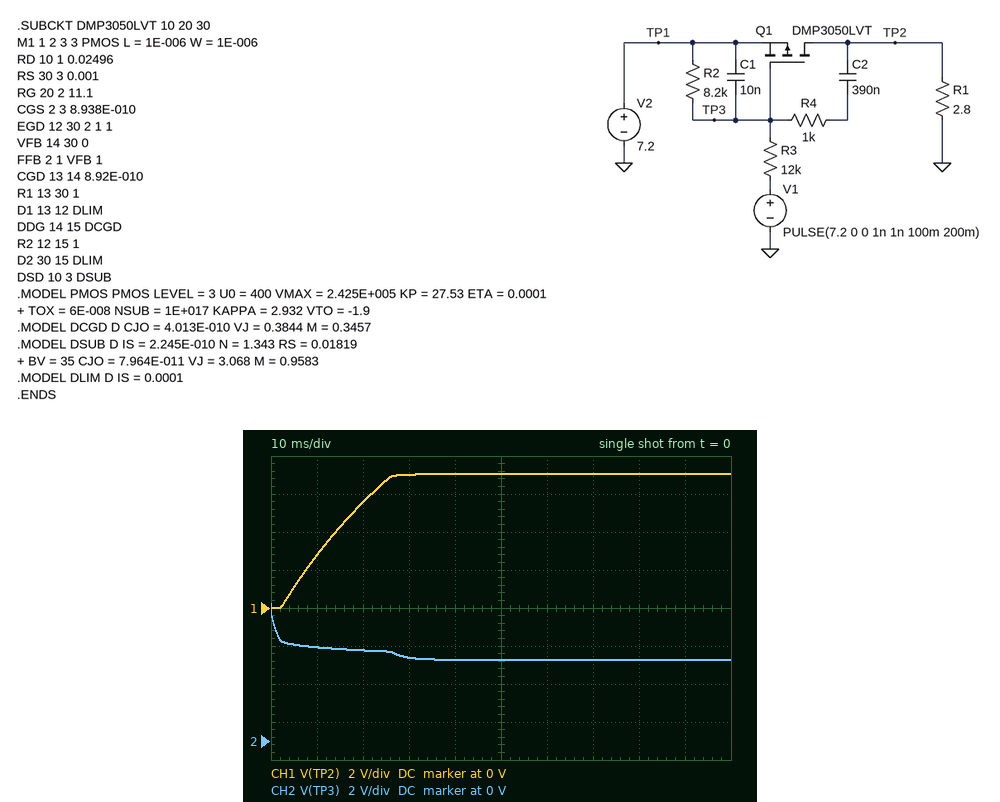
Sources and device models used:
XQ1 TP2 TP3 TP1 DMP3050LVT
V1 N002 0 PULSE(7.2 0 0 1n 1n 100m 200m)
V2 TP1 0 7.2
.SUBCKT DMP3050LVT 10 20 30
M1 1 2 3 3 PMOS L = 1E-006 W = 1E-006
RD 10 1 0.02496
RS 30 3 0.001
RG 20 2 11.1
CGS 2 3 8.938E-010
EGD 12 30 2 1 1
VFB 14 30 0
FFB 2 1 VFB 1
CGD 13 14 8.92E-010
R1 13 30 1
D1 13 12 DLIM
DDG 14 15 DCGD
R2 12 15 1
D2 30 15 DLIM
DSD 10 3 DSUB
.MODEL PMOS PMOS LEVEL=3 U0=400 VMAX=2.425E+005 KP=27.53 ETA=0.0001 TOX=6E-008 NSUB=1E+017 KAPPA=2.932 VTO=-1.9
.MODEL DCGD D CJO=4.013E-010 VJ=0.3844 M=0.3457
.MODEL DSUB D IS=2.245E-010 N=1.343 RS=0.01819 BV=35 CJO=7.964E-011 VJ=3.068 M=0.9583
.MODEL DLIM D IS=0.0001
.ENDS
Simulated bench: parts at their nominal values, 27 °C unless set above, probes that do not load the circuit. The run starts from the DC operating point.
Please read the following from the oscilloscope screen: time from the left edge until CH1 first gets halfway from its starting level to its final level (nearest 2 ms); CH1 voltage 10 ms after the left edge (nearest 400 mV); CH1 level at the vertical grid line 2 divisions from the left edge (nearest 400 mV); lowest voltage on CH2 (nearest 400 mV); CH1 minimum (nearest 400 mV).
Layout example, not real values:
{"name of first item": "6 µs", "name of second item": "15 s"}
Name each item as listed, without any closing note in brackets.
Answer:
{"time from the left edge until CH1 first gets halfway from its starting level to its final level": "12 ms", "CH1 voltage 10 ms after the left edge": "2.8 V", "CH1 level at the vertical grid line 2 divisions from the left edge": "5.6 V", "lowest voltage on CH2": "4.4 V", "CH1 minimum": "0 V"}
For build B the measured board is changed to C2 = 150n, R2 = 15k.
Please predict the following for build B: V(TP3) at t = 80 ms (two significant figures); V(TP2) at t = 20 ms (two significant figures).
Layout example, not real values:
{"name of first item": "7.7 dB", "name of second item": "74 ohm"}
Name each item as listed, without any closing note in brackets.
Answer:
{"V(TP3) at t = 80 ms": "3.2 V", "V(TP2) at t = 20 ms": "7.1 V"}
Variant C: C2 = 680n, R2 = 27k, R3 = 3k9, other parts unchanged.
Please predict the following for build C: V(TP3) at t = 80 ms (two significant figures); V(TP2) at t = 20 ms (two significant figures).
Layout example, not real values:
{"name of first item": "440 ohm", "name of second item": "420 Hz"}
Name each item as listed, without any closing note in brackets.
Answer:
{"V(TP3) at t = 80 ms": "910 mV", "V(TP2) at t = 20 ms": "7.1 V"}
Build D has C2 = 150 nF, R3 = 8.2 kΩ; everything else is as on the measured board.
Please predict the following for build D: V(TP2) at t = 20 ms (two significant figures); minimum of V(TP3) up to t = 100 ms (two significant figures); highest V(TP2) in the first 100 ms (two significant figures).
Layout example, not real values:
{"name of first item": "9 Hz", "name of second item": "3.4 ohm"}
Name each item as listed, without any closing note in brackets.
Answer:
{"V(TP2) at t = 20 ms": "7.1 V", "minimum of V(TP3) up to t = 100 ms": "3.6 V", "highest V(TP2) in the first 100 ms": "7.1 V"}
